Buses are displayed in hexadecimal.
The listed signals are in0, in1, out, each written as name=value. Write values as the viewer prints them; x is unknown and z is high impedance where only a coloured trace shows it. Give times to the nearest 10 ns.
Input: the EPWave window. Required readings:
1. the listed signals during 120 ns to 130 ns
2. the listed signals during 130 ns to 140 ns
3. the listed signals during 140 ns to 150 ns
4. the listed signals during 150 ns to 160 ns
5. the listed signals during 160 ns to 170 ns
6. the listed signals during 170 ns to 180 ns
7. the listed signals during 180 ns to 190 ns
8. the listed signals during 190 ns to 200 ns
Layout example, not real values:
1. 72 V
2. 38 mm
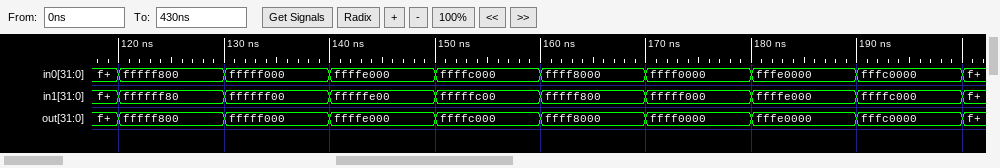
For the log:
1. in0=fffff800, in1=ffffff80, out=fffff800
2. in0=fffff000, in1=ffffff00, out=fffff000
3. in0=ffffe000, in1=fffffe00, out=ffffe000
4. in0=ffffc000, in1=fffffc00, out=ffffc000
5. in0=ffff8000, in1=fffff800, out=ffff8000
6. in0=ffff0000, in1=fffff000, out=ffff0000
7. in0=fffe0000, in1=ffffe000, out=fffe0000
8. in0=fffc0000, in1=ffffc000, out=fffc0000
